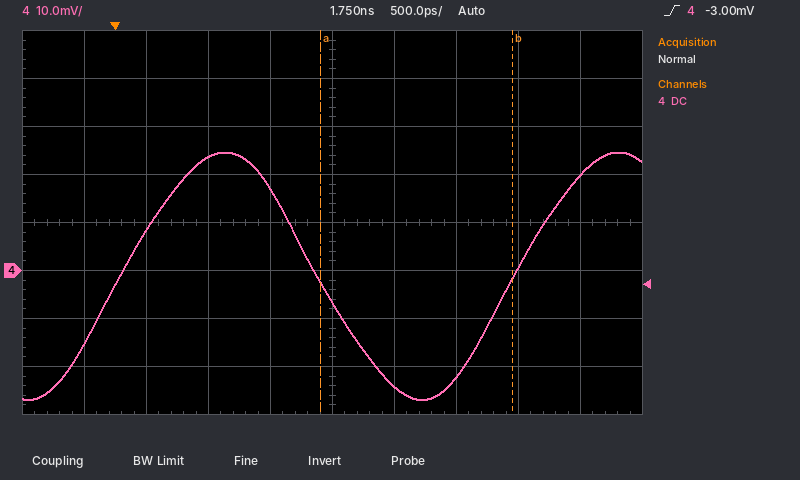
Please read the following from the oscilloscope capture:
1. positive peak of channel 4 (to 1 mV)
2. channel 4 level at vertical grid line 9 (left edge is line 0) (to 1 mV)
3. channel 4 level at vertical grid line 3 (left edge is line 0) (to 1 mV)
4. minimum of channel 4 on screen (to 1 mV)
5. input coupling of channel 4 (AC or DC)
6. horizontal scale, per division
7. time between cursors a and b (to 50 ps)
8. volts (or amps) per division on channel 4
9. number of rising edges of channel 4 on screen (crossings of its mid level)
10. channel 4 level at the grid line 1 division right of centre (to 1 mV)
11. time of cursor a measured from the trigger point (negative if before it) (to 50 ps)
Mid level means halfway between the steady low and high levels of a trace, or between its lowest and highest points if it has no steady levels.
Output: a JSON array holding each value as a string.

["25 mV", "20 mV", "24 mV", "-27 mV", "DC", "500 ps", "1.55 ns", "10 mV", "2", "-24 mV", "+1.65 ns"]
